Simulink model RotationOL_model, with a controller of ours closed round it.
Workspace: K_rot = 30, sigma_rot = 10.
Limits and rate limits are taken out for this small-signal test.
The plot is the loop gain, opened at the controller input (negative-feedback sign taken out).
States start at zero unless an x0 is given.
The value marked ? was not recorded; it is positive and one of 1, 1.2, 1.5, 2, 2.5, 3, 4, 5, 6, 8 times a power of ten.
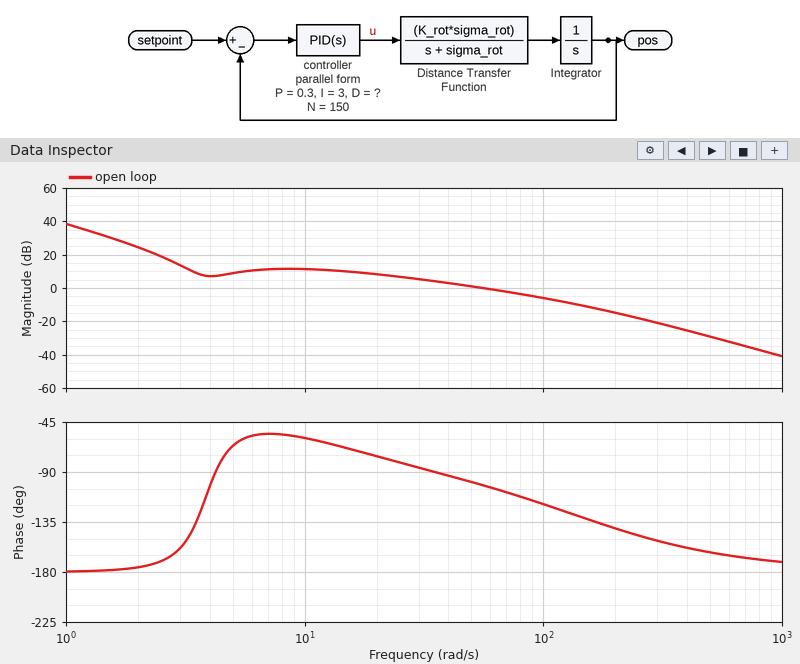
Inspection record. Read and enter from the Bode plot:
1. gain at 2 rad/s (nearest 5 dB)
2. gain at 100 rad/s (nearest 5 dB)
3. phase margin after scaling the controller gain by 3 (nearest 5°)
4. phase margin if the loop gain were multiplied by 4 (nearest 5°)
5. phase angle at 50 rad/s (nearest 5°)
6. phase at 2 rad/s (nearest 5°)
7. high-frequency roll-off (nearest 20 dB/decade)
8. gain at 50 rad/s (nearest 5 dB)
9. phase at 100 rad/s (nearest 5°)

25 dB
-5 dB
50°
45°
-100°
-175°
-40 dB/decade
0 dB
-120°
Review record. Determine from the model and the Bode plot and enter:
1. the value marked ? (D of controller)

0.2
